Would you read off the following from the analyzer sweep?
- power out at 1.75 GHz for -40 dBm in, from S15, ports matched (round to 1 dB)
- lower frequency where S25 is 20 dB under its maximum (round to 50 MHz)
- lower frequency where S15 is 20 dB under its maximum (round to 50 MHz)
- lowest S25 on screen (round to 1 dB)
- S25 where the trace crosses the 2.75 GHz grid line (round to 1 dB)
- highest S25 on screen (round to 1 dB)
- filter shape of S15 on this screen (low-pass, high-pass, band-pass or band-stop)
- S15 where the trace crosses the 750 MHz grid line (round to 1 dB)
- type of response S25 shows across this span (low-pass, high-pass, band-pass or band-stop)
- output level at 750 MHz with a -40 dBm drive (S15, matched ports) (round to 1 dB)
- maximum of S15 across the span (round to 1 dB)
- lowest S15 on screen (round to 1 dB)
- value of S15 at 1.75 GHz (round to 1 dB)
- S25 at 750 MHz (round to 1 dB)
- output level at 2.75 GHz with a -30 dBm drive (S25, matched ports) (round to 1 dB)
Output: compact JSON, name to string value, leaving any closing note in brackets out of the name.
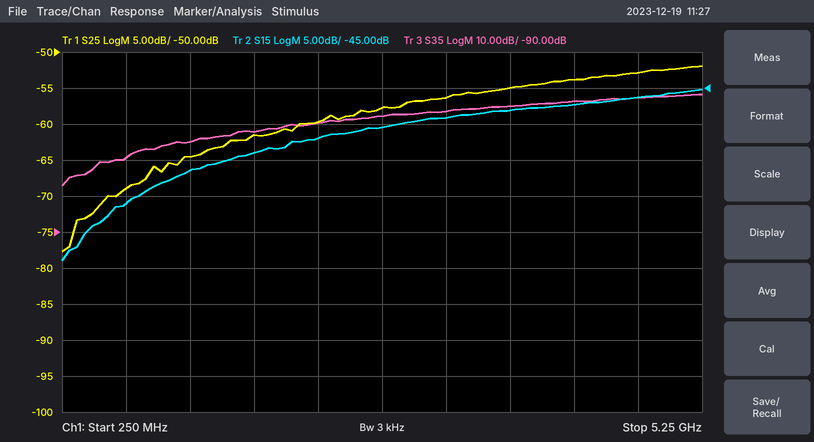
{"power out at 1.75 GHz for -40 dBm in, from S15, ports matched": "-94 dBm", "lower frequency where S25 is 20 dB under its maximum": "500 MHz", "lower frequency where S15 is 20 dB under its maximum": "450 MHz", "lowest S25 on screen": "-78 dB", "S25 where the trace crosses the 2.75 GHz grid line": "-58 dB", "highest S25 on screen": "-52 dB", "filter shape of S15 on this screen": "high-pass", "S15 where the trace crosses the 750 MHz grid line": "-61 dB", "type of response S25 shows across this span": "high-pass", "output level at 750 MHz with a -40 dBm drive (S15, matched ports)": "-101 dBm", "maximum of S15 across the span": "-45 dB", "lowest S15 on screen": "-69 dB", "value of S15 at 1.75 GHz": "-54 dB", "S25 at 750 MHz": "-69 dB", "output level at 2.75 GHz with a -30 dBm drive (S25, matched ports)": "-88 dBm"}
